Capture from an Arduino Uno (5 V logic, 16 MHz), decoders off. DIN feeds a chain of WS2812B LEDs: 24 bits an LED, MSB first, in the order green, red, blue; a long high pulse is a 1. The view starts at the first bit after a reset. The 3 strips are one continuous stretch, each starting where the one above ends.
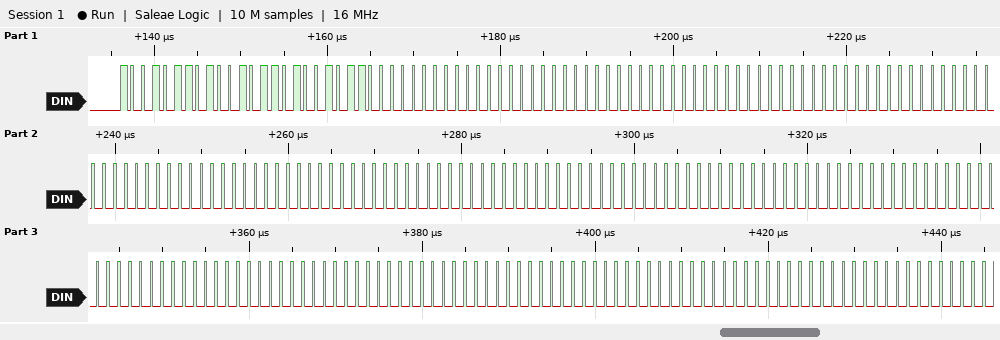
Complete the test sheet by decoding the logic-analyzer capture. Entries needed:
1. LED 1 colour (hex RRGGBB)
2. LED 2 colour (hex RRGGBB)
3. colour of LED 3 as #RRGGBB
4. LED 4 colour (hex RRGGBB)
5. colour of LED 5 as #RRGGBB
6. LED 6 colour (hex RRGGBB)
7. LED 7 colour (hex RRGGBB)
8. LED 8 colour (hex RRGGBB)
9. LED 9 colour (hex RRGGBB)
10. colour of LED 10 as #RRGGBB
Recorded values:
#969696
#000000
#000000
#000000
#000000
#000000
#000000
#000000
#000000
#000000
